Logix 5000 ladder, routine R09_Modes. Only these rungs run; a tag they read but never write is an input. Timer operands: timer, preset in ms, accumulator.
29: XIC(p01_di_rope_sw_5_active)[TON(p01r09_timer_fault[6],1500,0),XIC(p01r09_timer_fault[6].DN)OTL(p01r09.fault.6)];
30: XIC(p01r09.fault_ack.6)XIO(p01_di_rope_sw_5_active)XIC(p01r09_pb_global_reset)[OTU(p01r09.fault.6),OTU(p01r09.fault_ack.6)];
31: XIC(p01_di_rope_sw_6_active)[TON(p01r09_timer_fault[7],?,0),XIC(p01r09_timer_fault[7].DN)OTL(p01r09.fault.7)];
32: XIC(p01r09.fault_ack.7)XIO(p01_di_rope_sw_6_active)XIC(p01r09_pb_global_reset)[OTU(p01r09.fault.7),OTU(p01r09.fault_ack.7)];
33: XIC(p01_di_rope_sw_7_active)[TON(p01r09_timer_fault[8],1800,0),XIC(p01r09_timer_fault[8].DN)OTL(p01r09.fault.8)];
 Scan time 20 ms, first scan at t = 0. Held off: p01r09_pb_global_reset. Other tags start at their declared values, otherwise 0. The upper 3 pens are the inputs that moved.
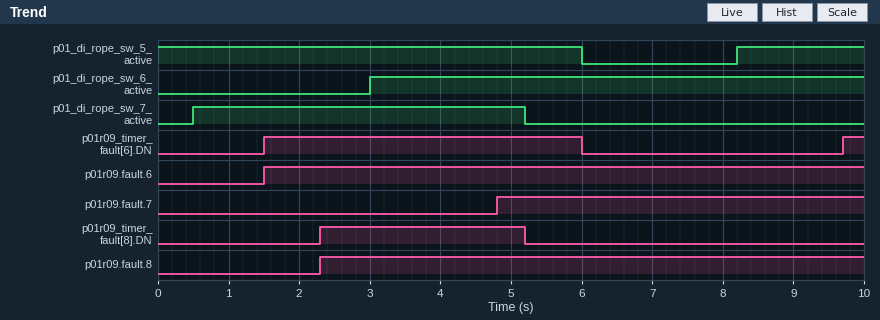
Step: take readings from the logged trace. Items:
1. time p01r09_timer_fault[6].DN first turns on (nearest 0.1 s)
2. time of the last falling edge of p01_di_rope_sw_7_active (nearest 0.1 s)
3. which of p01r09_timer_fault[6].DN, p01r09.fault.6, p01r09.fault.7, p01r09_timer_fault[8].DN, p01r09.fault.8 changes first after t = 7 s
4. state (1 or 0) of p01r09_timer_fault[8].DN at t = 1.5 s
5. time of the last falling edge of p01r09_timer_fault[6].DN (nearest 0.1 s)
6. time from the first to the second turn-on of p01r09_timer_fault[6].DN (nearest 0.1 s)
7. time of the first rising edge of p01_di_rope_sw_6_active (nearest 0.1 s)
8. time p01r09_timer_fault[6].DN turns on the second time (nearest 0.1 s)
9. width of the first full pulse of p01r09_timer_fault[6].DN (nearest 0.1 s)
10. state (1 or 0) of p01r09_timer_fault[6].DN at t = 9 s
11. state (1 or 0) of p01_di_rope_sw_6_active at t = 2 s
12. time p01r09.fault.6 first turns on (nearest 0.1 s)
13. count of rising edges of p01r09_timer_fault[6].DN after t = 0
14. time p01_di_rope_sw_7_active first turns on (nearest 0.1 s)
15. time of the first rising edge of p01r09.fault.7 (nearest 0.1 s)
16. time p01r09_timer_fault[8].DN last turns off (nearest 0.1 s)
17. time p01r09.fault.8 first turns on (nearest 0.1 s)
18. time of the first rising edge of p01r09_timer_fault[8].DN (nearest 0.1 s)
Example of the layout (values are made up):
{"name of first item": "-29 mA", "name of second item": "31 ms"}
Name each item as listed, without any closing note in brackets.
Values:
{"time p01r09_timer_fault[6].DN first turns on": "1.5 s", "time of the last falling edge of p01_di_rope_sw_7_active": "5.2 s", "which of p01r09_timer_fault[6].DN, p01r09.fault.6, p01r09.fault.7, p01r09_timer_fault[8].DN, p01r09.fault.8 changes first after t = 7 s": "p01r09_timer_fault[6].DN", "state (1 or 0) of p01r09_timer_fault[8].DN at t = 1.5 s": "0", "time of the last falling edge of p01r09_timer_fault[6].DN": "6.0 s", "time from the first to the second turn-on of p01r09_timer_fault[6].DN": "8.2 s", "time of the first rising edge of p01_di_rope_sw_6_active": "3.0 s", "time p01r09_timer_fault[6].DN turns on the second time": "9.7 s", "width of the first full pulse of p01r09_timer_fault[6].DN": "4.5 s", "state (1 or 0) of p01r09_timer_fault[6].DN at t = 9 s": "0", "state (1 or 0) of p01_di_rope_sw_6_active at t = 2 s": "0", "time p01r09.fault.6 first turns on": "1.5 s", "count of rising edges of p01r09_timer_fault[6].DN after t = 0": "2", "time p01_di_rope_sw_7_active first turns on": "0.5 s", "time of the first rising edge of p01r09.fault.7": "4.8 s", "time p01r09_timer_fault[8].DN last turns off": "5.2 s", "time p01r09.fault.8 first turns on": "2.3 s", "time of the first rising edge of p01r09_timer_fault[8].DN": "2.3 s"}
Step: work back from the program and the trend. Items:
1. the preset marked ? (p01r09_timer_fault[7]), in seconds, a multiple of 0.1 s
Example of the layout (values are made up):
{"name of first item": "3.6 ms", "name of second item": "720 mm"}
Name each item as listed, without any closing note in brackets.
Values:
{"the preset marked ? (p01r09_timer_fault[7]), in seconds, a multiple of 0.1 s": "1.8 s"}
